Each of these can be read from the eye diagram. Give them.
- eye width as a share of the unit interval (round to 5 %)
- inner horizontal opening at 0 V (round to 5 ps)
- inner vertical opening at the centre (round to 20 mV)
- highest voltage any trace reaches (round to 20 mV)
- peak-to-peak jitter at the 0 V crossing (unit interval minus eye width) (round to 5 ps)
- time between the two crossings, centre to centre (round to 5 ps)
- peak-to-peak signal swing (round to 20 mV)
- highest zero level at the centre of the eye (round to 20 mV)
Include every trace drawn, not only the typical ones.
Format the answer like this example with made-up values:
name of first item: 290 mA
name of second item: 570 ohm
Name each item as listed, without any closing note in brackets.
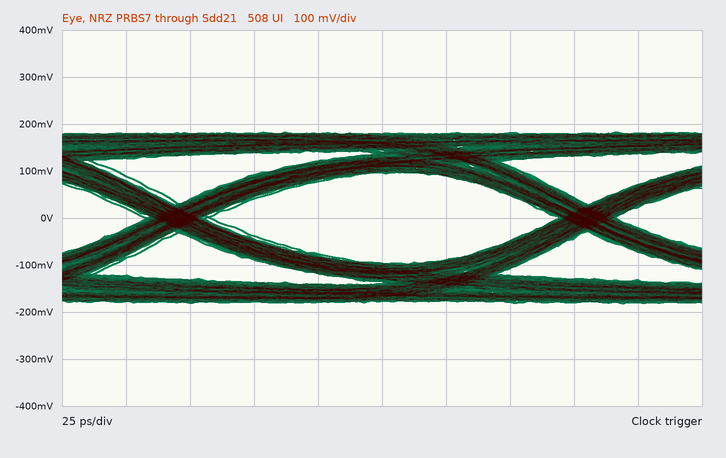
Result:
eye width as a share of the unit interval: 85 %
inner horizontal opening at 0 V: 135 ps
inner vertical opening at the centre: 200 mV
highest voltage any trace reaches: 180 mV
peak-to-peak jitter at the 0 V crossing (unit interval minus eye width): 25 ps
time between the two crossings, centre to centre: 160 ps
peak-to-peak signal swing: 360 mV
highest zero level at the centre of the eye: -100 mV
